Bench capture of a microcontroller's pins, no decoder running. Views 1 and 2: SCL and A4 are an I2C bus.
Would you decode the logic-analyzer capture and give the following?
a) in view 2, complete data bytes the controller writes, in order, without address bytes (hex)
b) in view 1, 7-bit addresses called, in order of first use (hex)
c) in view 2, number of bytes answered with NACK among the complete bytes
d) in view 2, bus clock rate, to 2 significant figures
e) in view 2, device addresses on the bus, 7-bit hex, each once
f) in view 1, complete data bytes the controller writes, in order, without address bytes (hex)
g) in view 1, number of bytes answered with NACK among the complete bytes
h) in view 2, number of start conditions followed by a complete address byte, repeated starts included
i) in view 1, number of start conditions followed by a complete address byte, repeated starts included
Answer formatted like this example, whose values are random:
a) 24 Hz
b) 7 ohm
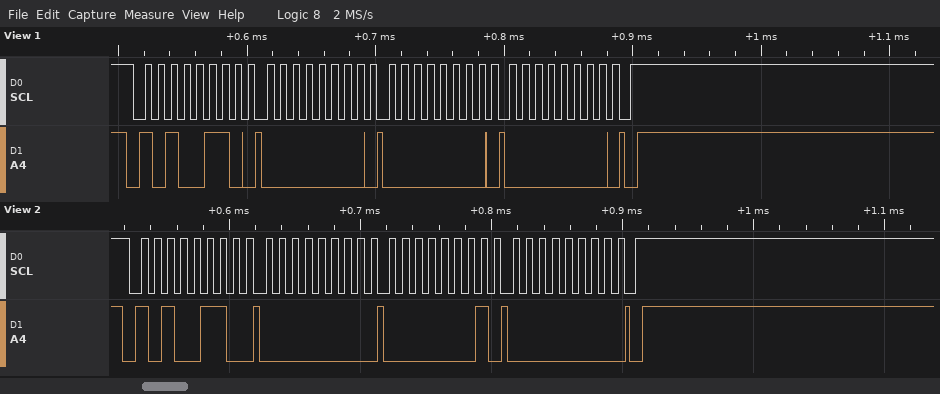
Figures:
a) 00 01 00
b) 0x53
c) 0
d) 100 kHz
e) 0x53
f) 00 00 00
g) 0
h) 1
i) 1
